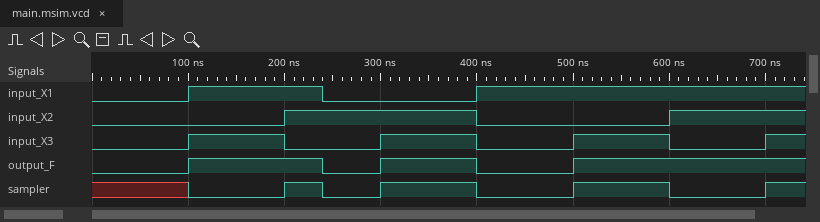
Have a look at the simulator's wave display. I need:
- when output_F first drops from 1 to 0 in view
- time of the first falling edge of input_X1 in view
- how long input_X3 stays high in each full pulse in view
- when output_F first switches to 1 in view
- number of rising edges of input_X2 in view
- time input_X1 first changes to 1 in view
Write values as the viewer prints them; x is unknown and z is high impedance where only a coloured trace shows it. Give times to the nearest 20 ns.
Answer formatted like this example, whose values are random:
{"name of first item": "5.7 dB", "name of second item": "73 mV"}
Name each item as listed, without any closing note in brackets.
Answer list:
{"when output_F first drops from 1 to 0 in view": "240 ns", "time of the first falling edge of input_X1 in view": "240 ns", "how long input_X3 stays high in each full pulse in view": "100 ns, 100 ns, 100 ns", "when output_F first switches to 1 in view": "100 ns", "number of rising edges of input_X2 in view": "2", "time input_X1 first changes to 1 in view": "100 ns"}
